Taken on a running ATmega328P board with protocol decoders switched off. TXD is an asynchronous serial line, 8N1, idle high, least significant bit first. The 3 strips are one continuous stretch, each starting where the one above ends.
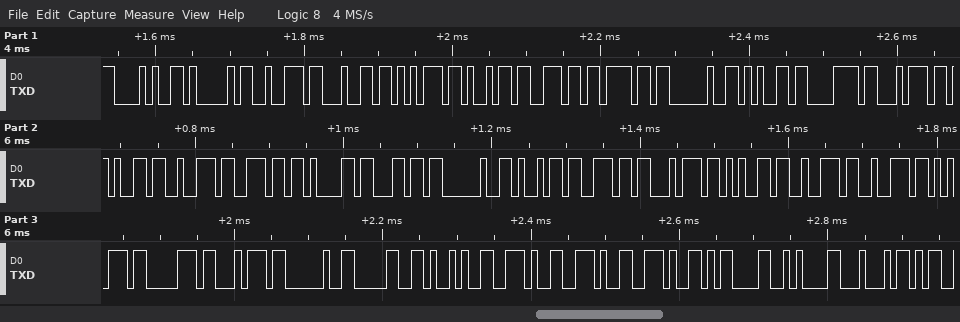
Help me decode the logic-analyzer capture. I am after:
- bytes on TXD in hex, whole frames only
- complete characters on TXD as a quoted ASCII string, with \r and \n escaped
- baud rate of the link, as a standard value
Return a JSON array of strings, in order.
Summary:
["0x28 0x41 0x72 0x64 0x75 0x69 0x6E 0x6F 0x20 0x65 0x78 0x74 0x65 0x72 0x6E 0x61 0x6C 0x20 0x69 0x6E 0x74 0x65 0x72 0x72 0x75 0x70 0x74 0x20 0x30 0x29 0x2E 0x2E 0x2E 0x0D 0x0A 0x44", "\"(Arduino external interrupt 0)...\\r\\nD\"", "115200 baud"]
